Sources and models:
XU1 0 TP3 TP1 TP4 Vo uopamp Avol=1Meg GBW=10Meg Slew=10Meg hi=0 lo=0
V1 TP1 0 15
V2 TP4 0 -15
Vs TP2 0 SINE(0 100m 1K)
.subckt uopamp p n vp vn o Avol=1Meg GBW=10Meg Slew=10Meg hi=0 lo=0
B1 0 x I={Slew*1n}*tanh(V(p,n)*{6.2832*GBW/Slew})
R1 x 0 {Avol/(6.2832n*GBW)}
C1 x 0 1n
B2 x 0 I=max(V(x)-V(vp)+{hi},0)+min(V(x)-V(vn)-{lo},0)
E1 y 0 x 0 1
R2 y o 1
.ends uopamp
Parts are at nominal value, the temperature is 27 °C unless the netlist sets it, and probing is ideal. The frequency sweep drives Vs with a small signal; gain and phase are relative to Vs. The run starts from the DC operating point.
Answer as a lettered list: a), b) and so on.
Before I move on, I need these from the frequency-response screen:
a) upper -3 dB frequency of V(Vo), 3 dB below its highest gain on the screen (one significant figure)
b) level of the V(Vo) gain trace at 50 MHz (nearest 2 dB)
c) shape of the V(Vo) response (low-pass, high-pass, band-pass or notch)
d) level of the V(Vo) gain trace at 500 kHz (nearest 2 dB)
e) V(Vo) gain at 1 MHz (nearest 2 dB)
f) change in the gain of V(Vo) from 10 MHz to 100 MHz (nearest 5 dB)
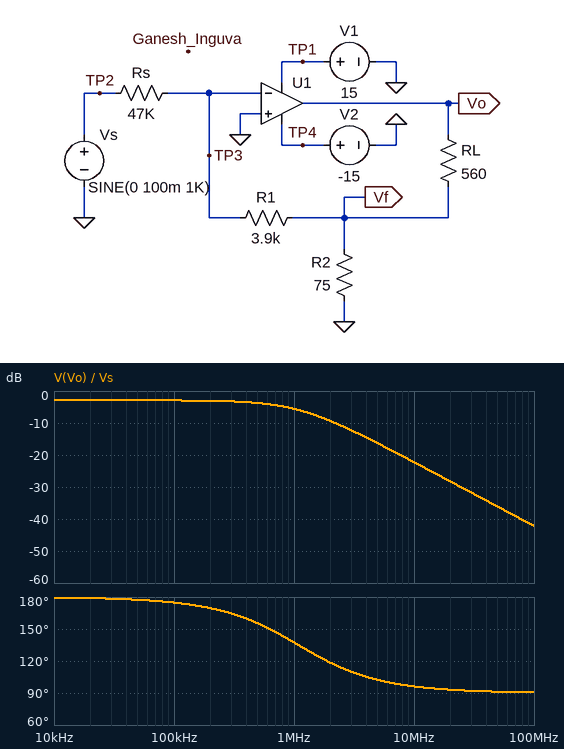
a) 1 MHz
b) -36 dB
c) low-pass
d) -4 dB
e) -6 dB
f) -20 dB
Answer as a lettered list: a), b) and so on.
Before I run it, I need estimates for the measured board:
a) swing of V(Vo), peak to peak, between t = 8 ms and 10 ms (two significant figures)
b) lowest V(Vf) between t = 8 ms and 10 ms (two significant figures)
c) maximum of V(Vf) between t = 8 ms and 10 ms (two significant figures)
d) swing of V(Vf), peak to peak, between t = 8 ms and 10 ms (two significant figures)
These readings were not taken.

a) 140 mV
b) -8.3 mV
c) 8.3 mV
d) 17 mV
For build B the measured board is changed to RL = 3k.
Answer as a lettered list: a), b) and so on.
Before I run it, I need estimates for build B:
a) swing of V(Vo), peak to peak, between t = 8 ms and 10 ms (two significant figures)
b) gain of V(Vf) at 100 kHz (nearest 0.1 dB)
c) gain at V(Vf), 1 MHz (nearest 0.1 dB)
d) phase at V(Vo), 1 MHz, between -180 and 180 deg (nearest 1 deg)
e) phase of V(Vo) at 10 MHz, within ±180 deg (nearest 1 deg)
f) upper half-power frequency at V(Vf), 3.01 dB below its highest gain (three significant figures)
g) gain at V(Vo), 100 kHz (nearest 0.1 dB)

a) 690 mV
b) -22.4 dB
c) -34.8 dB
d) 103 deg
e) 91 deg
f) 225 kHz
g) 10.0 dB
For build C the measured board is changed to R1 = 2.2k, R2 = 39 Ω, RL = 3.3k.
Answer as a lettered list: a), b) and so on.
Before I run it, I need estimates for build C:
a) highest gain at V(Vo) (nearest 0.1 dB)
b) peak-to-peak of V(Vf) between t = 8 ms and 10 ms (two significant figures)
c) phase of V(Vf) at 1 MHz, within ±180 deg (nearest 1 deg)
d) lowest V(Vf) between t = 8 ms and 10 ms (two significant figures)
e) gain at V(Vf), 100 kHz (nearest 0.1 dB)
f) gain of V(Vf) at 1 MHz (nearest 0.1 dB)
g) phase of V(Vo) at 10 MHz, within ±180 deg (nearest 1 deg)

a) 12.2 dB
b) 9.4 mV
c) 88 deg
d) -4.7 mV
e) -29.2 dB
f) -45.6 dB
g) 91 deg
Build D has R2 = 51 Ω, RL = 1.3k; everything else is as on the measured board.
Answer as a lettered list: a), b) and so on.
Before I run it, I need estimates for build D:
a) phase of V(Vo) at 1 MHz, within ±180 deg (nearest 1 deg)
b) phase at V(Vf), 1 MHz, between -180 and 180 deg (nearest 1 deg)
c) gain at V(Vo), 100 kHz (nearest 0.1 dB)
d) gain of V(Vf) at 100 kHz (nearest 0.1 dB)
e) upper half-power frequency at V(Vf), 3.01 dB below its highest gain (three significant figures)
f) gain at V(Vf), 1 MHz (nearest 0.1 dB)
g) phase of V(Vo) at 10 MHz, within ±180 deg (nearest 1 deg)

a) 109 deg
b) 107 deg
c) 6.6 dB
d) -22.0 dB
e) 348 kHz
f) -31.3 dB
g) 92 deg
